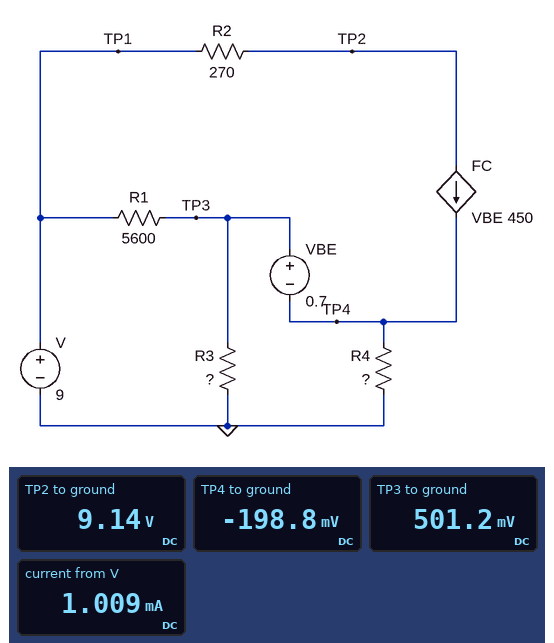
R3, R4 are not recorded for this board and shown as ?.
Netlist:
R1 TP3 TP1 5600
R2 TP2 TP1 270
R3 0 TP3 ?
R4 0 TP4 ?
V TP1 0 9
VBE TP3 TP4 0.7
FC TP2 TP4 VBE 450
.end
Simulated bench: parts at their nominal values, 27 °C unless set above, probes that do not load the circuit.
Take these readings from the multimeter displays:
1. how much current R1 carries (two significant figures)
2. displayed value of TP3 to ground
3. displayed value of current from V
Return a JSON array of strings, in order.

["1.5 mA", "501.2 mV", "1.009 mA"]
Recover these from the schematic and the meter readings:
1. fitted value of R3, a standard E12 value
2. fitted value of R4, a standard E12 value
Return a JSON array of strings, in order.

["330 Ω", "390 Ω"]
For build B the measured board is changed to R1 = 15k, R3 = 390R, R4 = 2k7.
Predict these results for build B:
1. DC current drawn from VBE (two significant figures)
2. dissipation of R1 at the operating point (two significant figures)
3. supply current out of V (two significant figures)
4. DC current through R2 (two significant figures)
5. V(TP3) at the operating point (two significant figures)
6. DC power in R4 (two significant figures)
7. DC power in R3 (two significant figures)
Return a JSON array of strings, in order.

["390 nA", "5.1 mW", "410 µA", "170 µA", "230 mV", "82 µW", "130 µW"]
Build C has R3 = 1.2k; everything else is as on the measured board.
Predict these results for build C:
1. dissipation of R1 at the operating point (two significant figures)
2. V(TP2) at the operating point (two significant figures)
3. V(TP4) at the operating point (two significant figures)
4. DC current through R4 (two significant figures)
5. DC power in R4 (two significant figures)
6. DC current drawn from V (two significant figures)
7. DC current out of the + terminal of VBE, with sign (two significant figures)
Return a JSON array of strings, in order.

["9.8 mW", "8.4 V", "880 mV", "2.3 mA", "2.0 mW", "3.6 mA", "-5.0 µA"]
